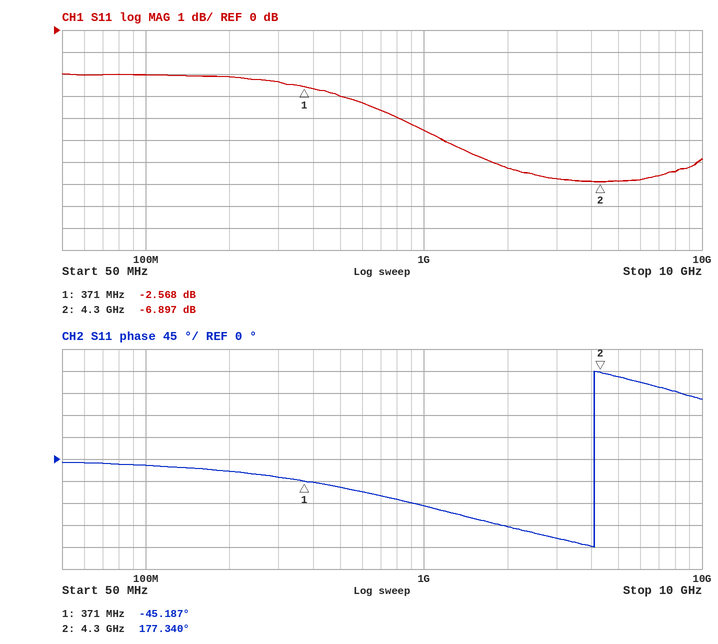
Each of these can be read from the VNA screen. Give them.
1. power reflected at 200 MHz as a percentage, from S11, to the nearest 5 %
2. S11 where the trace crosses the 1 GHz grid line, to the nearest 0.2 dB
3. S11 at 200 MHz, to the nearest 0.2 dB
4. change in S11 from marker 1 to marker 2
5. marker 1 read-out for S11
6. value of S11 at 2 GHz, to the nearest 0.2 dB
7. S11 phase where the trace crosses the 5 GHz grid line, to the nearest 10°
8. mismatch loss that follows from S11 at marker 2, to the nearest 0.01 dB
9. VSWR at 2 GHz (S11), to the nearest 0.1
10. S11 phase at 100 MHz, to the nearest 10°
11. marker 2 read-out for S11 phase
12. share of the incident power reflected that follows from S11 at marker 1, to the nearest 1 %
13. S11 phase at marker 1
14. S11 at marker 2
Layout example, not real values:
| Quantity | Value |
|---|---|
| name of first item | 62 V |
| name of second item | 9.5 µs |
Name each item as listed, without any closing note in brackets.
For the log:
| Quantity | Value |
|---|---|
| power reflected at 200 MHz as a percentage, from S11, to the nearest 5 % | 60 % |
| S11 where the trace crosses the 1 GHz grid line, to the nearest 0.2 dB | -4.6 dB |
| S11 at 200 MHz, to the nearest 0.2 dB | -2.2 dB |
| change in S11 from marker 1 to marker 2 | -4.329 dB |
| marker 1 read-out for S11 | -2.568 dB |
| value of S11 at 2 GHz, to the nearest 0.2 dB | -6.2 dB |
| S11 phase where the trace crosses the 5 GHz grid line, to the nearest 10° | 170° |
| mismatch loss that follows from S11 at marker 2, to the nearest 0.01 dB | 0.99 dB |
| VSWR at 2 GHz (S11), to the nearest 0.1 | 2.9 |
| S11 phase at 100 MHz, to the nearest 10° | -10° |
| marker 2 read-out for S11 phase | 177.340° |
| share of the incident power reflected that follows from S11 at marker 1, to the nearest 1 % | 55 % |
| S11 phase at marker 1 | -45.187° |
| S11 at marker 2 | -6.897 dB |
